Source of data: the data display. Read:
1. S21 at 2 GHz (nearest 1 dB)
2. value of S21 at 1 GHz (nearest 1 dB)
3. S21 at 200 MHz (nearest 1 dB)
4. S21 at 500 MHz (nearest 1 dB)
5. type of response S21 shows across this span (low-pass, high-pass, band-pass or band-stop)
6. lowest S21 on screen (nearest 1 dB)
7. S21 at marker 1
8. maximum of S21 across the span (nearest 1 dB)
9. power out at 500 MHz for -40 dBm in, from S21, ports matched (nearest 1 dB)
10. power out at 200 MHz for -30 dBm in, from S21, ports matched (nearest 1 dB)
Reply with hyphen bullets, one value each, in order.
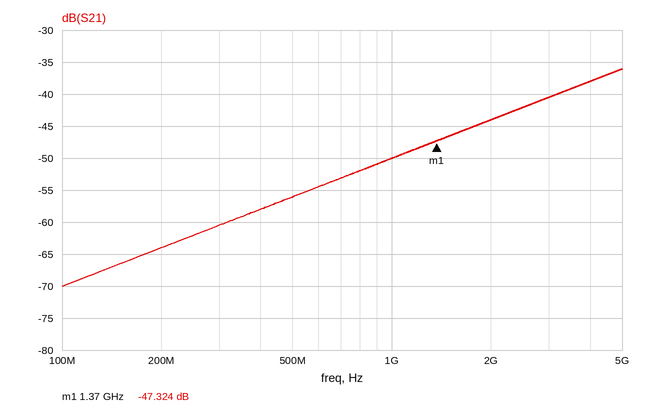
- -44 dB
- -50 dB
- -64 dB
- -56 dB
- high-pass
- -70 dB
- -47.324 dB
- -36 dB
- -96 dBm
- -94 dBm
